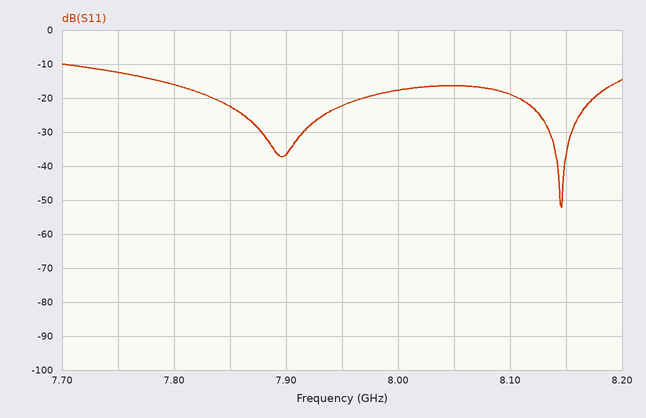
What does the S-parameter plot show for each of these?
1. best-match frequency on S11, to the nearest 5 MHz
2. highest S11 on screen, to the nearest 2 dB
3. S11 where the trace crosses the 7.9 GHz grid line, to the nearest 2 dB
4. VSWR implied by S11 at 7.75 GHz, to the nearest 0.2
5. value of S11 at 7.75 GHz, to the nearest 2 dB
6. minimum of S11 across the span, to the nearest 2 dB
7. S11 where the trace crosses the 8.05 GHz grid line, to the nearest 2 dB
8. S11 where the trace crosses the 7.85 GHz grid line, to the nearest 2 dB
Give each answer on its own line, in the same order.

8.145 GHz
-10 dB
-36 dB
1.6
-12 dB
-52 dB
-16 dB
-22 dB
